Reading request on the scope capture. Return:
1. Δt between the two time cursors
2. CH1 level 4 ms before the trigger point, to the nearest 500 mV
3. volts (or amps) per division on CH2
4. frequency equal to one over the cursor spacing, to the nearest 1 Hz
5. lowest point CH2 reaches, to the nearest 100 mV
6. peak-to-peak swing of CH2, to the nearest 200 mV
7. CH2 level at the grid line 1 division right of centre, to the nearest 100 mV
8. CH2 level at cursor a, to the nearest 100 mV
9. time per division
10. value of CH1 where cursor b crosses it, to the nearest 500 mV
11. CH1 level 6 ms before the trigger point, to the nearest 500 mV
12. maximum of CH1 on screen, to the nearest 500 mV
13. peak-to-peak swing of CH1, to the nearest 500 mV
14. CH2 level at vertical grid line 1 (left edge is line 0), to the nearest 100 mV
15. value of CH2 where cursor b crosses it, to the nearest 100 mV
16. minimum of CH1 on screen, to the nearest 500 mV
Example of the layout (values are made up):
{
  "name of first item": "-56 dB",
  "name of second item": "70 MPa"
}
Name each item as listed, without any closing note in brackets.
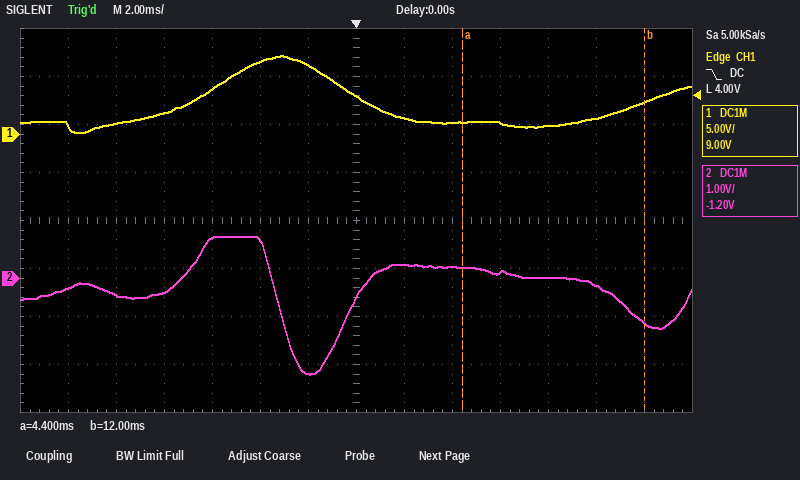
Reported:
{
  "Δt between the two time cursors": "7.6 ms",
  "CH1 level 4 ms before the trigger point, to the nearest 500 mV": "7.5 V",
  "volts (or amps) per division on CH2": "1 V",
  "frequency equal to one over the cursor spacing, to the nearest 1 Hz": "132 Hz",
  "lowest point CH2 reaches, to the nearest 100 mV": "-2.0 V",
  "peak-to-peak swing of CH2, to the nearest 200 mV": "2.8 V",
  "CH2 level at the grid line 1 division right of centre, to the nearest 100 mV": "300 mV",
  "CH2 level at cursor a, to the nearest 100 mV": "200 mV",
  "time per division": "2 ms",
  "value of CH1 where cursor b crosses it, to the nearest 500 mV": "3.5 V",
  "CH1 level 6 ms before the trigger point, to the nearest 500 mV": "4.5 V",
  "maximum of CH1 on screen, to the nearest 500 mV": "8.0 V",
  "peak-to-peak swing of CH1, to the nearest 500 mV": "8.0 V",
  "CH2 level at vertical grid line 1 (left edge is line 0), to the nearest 100 mV": "-200 mV",
  "value of CH2 where cursor b crosses it, to the nearest 100 mV": "-900 mV",
  "minimum of CH1 on screen, to the nearest 500 mV": "0.0 V"
}
